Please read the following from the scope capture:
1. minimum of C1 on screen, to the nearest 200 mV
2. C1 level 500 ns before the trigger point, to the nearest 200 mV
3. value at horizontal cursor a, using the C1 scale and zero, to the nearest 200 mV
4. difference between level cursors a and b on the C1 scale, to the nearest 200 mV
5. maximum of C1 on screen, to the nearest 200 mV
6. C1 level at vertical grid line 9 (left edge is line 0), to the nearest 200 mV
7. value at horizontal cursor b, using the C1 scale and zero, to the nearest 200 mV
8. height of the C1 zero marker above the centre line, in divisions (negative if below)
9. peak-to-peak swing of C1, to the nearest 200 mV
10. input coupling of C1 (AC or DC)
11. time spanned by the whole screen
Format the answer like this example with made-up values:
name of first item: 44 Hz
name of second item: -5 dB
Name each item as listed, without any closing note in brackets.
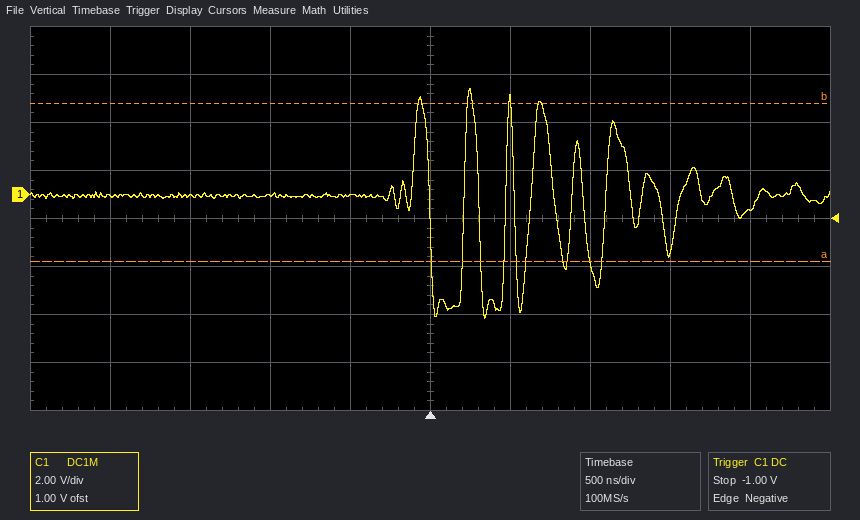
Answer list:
minimum of C1 on screen, to the nearest 200 mV: -5.2 V
C1 level 500 ns before the trigger point, to the nearest 200 mV: 0.0 V
value at horizontal cursor a, using the C1 scale and zero, to the nearest 200 mV: -2.8 V
difference between level cursors a and b on the C1 scale, to the nearest 200 mV: 6.6 V
maximum of C1 on screen, to the nearest 200 mV: 4.4 V
C1 level at vertical grid line 9 (left edge is line 0), to the nearest 200 mV: -600 mV
value at horizontal cursor b, using the C1 scale and zero, to the nearest 200 mV: 3.8 V
height of the C1 zero marker above the centre line, in divisions: +0.5 div
peak-to-peak swing of C1, to the nearest 200 mV: 9.6 V
input coupling of C1: DC
time spanned by the whole screen: 5 µs
